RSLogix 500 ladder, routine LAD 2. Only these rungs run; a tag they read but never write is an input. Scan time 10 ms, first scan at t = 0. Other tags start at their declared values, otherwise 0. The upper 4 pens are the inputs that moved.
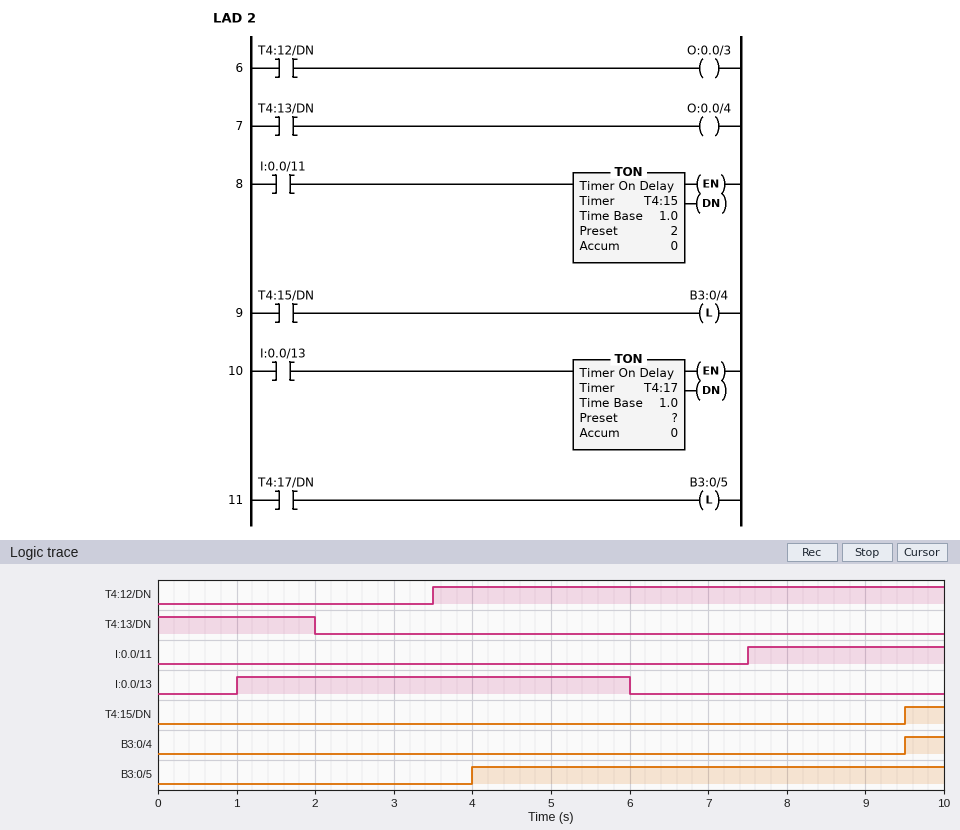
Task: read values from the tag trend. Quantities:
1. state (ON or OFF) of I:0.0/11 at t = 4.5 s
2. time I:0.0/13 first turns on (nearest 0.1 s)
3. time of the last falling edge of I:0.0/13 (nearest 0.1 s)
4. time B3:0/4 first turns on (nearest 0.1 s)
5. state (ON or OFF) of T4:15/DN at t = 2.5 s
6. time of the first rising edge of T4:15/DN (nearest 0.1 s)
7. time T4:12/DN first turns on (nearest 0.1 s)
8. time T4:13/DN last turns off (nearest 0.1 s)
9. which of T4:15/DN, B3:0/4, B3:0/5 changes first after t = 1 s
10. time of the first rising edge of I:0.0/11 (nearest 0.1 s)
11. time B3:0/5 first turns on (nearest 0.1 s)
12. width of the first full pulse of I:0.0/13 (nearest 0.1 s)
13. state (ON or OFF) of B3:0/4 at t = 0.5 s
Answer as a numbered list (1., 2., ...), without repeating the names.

1. OFF
2. 1.0 s
3. 6.0 s
4. 9.5 s
5. OFF
6. 9.5 s
7. 3.5 s
8. 2.0 s
9. B3:0/5
10. 7.5 s
11. 4.0 s
12. 5.0 s
13. OFF
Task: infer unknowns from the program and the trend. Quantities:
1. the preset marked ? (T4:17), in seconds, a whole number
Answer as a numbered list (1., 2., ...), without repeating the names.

1. 3 s
